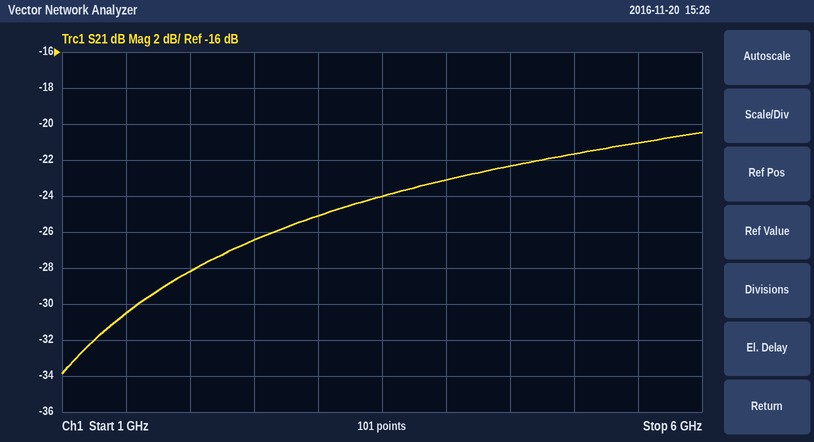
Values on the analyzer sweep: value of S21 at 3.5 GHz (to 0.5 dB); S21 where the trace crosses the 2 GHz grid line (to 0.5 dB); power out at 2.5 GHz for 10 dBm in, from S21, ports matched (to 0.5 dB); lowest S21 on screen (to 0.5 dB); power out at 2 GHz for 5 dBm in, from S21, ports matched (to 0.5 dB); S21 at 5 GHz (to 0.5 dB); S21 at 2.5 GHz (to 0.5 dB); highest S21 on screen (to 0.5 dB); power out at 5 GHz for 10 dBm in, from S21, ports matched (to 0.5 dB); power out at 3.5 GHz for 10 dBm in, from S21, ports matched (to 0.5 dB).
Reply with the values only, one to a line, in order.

-24.0 dB
-28.0 dB
-16.5 dBm
-34.0 dB
-23.0 dBm
-21.5 dB
-26.5 dB
-20.5 dB
-11.5 dBm
-14.0 dBm
